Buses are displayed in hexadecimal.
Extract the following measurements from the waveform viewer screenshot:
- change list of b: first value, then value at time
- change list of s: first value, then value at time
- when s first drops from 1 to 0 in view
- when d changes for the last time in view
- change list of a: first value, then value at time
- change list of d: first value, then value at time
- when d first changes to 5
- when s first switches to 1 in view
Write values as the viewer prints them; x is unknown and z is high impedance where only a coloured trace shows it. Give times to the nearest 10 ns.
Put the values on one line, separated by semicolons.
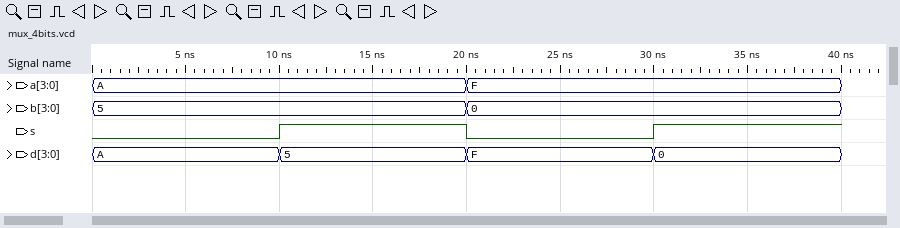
5, 0 at 20 ns; 0, 1 at 10 ns, 0 at 20 ns, 1 at 30 ns; 20 ns; 30 ns; A, F at 20 ns; A, 5 at 10 ns, F at 20 ns, 0 at 30 ns; 10 ns; 10 ns
